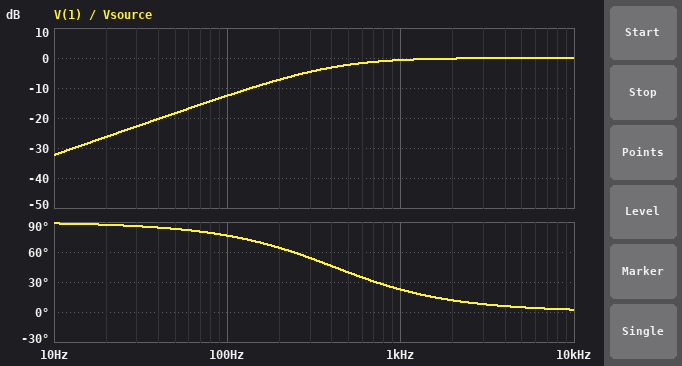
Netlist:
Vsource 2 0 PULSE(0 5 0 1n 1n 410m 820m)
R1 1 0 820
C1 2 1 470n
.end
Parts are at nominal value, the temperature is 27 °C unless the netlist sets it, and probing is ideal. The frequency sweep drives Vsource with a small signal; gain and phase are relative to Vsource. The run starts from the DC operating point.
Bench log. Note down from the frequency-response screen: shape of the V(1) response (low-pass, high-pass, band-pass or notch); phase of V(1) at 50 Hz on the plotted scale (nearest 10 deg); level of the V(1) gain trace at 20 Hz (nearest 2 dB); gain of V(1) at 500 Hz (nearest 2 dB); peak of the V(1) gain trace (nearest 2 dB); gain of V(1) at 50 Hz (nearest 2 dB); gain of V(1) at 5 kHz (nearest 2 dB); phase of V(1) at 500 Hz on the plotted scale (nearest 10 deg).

high-pass
80 deg
-26 dB
-2 dB
0 dB
-18 dB
0 dB
40 deg
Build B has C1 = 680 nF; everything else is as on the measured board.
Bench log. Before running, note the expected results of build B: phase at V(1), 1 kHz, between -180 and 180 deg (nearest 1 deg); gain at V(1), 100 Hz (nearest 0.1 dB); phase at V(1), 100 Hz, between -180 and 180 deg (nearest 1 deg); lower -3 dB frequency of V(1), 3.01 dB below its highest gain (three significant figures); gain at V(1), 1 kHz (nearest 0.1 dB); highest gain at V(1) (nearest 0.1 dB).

16 deg
-9.6 dB
71 deg
285 Hz
-0.3 dB
0 dB
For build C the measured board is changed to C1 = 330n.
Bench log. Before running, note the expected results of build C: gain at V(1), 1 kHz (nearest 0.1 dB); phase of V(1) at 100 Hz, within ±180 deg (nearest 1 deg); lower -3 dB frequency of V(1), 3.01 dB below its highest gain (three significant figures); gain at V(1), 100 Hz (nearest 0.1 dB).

-1.3 dB
80 deg
588 Hz
-15.5 dB
